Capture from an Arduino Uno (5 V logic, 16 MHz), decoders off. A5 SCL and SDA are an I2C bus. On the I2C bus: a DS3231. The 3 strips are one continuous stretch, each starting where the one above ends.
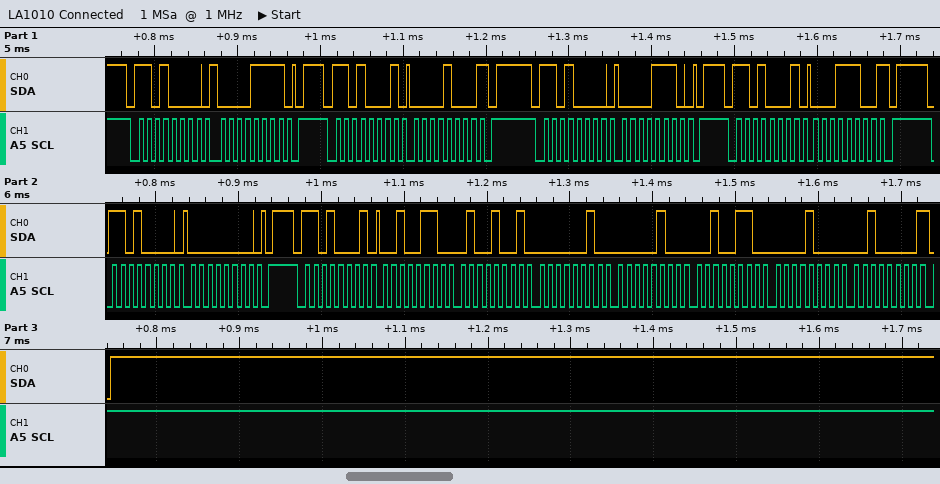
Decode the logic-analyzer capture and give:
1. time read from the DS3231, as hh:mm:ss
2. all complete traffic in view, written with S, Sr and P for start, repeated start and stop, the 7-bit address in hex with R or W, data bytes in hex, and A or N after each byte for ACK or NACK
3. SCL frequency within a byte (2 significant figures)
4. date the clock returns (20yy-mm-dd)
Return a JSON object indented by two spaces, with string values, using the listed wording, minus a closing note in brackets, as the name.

{
  "time read from the DS3231, as hh:mm:ss": "02:49:26",
  "all complete traffic in view, written with S, Sr and P for start, repeated start and stop, the 7-bit address in hex with R or W, data bytes in hex, and A or N after each byte for ACK or NACK": "S 68W A 0F A P S 68R A 08 N P S 68W A 0E A P S 68R A 1C N P S 68W A 00 A P S 68R A 26 A 49 A 02 A 04 A 26 A 08 A 20 N P",
  "SCL frequency within a byte": "100 kHz",
  "date the clock returns": "2020-08-26"
}
